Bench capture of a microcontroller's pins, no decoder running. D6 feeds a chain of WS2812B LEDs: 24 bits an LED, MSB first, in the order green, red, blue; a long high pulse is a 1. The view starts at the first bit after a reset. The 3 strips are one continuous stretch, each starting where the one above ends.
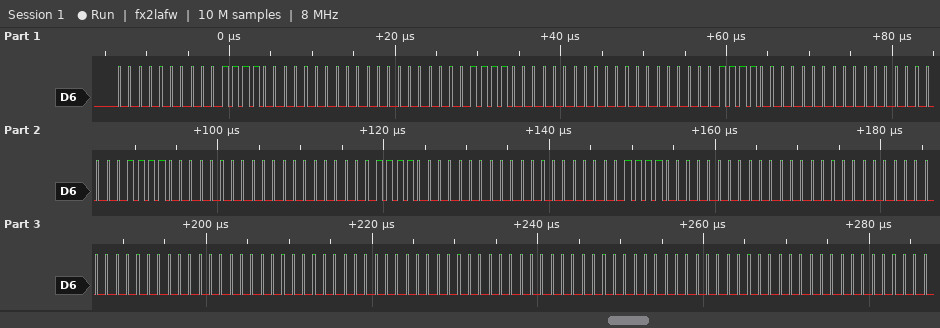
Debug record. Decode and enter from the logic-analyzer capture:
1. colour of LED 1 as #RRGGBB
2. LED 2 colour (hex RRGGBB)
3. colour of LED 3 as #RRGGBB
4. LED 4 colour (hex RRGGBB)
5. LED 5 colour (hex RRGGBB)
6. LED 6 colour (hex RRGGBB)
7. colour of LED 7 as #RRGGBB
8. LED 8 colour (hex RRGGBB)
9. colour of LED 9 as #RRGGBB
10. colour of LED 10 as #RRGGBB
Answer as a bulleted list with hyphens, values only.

- #3C0000
- #3C0000
- #3C0000
- #3C0000
- #3C0000
- #3C0000
- #000000
- #000000
- #000000
- #000000
